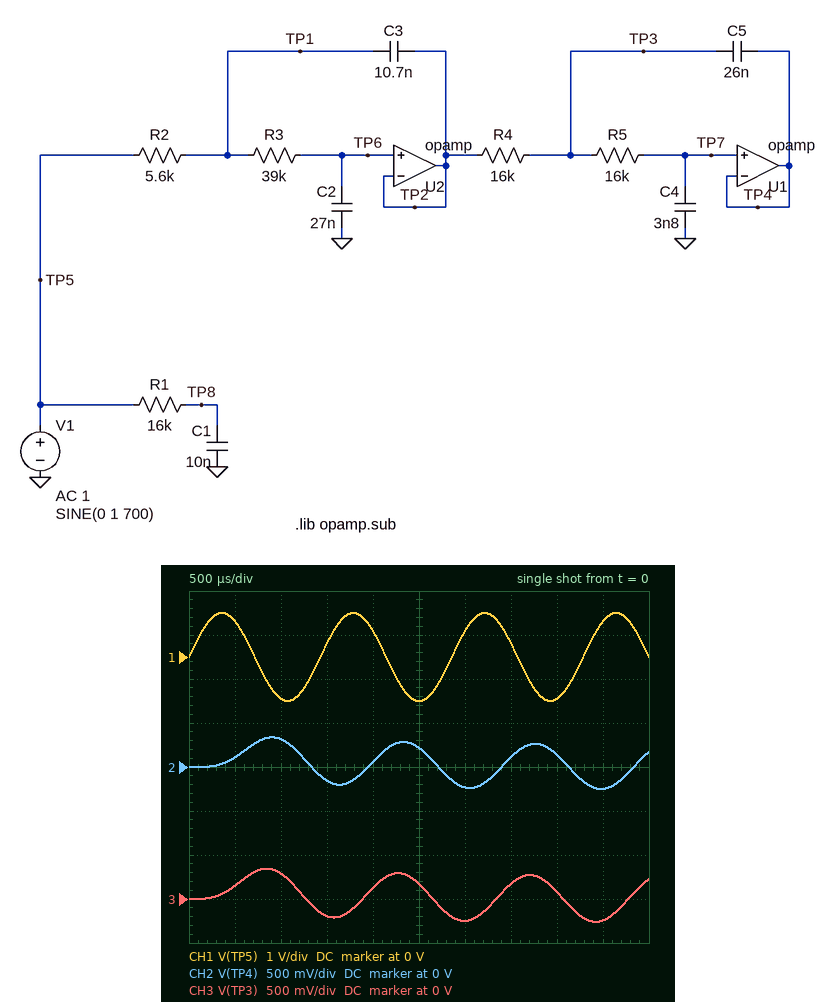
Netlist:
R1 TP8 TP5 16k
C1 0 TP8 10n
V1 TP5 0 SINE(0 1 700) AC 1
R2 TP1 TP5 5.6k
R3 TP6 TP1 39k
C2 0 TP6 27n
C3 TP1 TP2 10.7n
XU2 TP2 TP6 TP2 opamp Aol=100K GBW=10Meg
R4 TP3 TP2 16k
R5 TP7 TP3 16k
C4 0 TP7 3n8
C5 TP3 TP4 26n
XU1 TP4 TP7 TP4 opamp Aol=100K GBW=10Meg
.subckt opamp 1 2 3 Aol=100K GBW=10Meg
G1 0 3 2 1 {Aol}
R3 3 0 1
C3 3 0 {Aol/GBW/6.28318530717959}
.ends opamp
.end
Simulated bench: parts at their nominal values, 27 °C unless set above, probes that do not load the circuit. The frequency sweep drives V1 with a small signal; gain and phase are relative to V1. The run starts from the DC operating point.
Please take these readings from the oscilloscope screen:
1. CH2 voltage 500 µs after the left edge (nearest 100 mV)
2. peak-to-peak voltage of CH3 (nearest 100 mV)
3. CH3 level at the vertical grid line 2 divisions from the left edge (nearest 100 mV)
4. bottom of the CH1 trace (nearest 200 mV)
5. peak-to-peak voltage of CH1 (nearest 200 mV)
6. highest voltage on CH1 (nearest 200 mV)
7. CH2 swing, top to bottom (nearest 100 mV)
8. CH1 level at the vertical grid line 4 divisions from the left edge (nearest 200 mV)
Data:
100 mV
600 mV
300 mV
-1.0 V
2.0 V
1.0 V
600 mV
600 mV
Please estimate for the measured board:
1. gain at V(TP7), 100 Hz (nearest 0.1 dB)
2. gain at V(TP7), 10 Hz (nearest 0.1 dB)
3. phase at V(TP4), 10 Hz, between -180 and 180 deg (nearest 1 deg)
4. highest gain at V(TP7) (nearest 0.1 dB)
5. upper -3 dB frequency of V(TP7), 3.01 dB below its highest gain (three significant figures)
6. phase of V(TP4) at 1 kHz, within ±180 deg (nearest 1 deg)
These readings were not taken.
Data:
-1.8 dB
0 dB
-5 deg
0 dB
142 Hz
169 deg
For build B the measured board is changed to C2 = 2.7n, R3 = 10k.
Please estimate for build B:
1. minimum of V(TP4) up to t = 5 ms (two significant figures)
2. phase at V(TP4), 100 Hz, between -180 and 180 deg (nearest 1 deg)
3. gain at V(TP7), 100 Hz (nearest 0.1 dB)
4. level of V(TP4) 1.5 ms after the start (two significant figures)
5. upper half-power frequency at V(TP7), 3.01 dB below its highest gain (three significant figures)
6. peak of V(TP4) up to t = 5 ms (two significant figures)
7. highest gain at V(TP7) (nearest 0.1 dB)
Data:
-1.4 V
-6 deg
0.1 dB
-890 mV
1.20 kHz
1.4 V
3.2 dB
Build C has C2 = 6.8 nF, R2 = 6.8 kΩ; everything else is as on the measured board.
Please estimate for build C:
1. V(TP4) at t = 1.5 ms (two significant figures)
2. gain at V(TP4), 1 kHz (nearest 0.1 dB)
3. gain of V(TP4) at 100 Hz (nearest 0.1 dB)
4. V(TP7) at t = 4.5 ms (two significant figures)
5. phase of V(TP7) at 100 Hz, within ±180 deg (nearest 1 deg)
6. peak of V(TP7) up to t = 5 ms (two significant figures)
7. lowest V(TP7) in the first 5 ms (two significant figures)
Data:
-880 mV
-3.6 dB
0 dB
-760 mV
-16 deg
900 mV
-900 mV
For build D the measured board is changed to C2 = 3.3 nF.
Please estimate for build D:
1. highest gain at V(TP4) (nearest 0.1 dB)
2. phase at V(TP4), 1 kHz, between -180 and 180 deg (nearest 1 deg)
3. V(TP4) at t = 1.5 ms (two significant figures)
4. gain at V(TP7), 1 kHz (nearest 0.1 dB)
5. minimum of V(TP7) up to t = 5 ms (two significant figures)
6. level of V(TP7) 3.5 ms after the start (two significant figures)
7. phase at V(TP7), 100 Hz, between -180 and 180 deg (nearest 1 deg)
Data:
2.2 dB
-143 deg
-1.2 V
1.1 dB
-1.3 V
1.2 V
-10 deg
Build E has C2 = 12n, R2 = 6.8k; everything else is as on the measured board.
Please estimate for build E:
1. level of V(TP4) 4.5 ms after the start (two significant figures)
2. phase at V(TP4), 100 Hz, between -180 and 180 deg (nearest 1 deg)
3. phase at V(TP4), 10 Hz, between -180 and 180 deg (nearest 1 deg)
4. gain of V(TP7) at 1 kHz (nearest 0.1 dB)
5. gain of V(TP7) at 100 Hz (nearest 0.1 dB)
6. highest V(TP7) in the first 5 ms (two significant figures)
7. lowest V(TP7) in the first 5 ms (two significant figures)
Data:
-530 mV
-24 deg
-2 deg
-8.5 dB
-0.3 dB
590 mV
-550 mV
